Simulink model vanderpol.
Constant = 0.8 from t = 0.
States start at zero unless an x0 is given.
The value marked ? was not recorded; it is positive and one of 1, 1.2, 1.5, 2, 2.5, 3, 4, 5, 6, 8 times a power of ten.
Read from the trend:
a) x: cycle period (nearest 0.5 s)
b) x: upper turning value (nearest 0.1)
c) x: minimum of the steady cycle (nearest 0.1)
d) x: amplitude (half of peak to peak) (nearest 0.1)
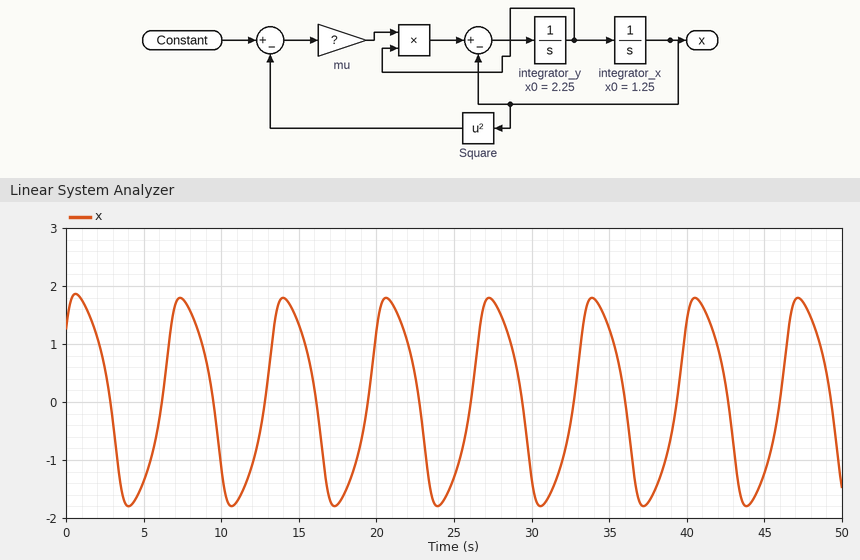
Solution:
6.5 s
1.8
-1.8
1.8
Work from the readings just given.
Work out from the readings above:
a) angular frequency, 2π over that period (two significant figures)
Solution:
0.97 rad/s
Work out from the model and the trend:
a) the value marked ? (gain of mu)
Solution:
1.2
